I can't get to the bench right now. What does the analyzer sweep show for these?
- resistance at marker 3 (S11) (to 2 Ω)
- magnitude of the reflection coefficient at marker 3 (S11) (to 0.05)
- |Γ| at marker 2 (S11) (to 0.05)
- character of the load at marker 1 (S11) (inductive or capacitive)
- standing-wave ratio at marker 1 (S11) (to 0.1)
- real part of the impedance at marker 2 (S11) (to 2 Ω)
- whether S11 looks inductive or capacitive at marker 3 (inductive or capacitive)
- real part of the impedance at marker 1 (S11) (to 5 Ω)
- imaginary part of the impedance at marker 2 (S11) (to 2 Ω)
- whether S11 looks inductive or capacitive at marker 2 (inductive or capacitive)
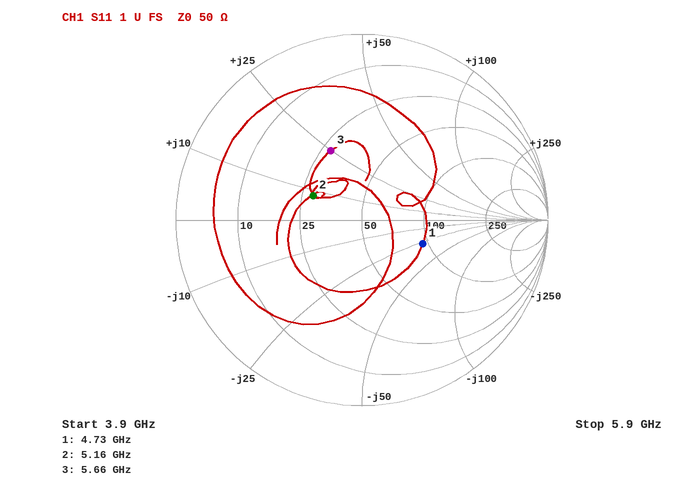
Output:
28 Ω
0.40
0.30
capacitive
2.1
28 Ω
inductive
95 Ω
+8 Ω
inductive
